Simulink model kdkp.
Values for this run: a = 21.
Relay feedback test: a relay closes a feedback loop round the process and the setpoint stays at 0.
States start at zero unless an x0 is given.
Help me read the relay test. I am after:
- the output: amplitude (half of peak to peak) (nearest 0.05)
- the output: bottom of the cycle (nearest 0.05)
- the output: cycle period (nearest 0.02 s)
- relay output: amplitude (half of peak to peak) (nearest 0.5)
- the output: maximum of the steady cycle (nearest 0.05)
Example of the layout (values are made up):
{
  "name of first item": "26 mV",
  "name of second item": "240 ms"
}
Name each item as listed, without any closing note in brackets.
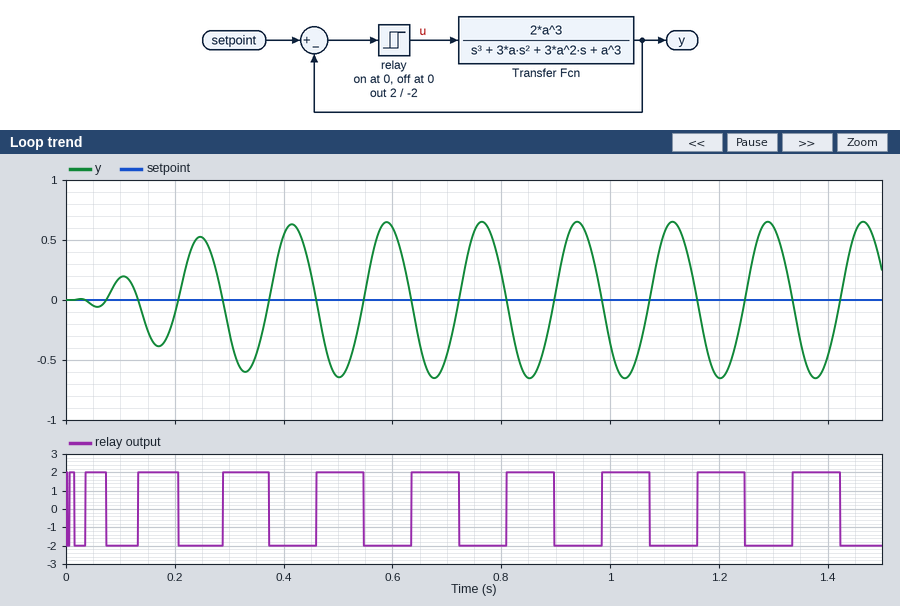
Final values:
{
  "the output: amplitude (half of peak to peak)": "0.65",
  "the output: bottom of the cycle": "-0.65",
  "the output: cycle period": "0.18 s",
  "relay output: amplitude (half of peak to peak)": "2.0",
  "the output: maximum of the steady cycle": "0.65"
}
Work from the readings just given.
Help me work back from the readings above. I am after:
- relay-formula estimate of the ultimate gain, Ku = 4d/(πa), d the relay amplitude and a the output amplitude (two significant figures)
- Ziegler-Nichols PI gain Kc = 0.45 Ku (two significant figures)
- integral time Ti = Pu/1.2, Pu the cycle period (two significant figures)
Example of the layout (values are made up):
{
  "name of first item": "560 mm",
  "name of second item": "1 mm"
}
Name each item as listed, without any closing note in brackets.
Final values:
{
  "relay-formula estimate of the ultimate gain, Ku = 4d/(πa), d the relay amplitude and a the output amplitude": "3.9",
  "Ziegler-Nichols PI gain Kc = 0.45 Ku": "1.8",
  "integral time Ti = Pu/1.2, Pu the cycle period": "0.15 s"
}
